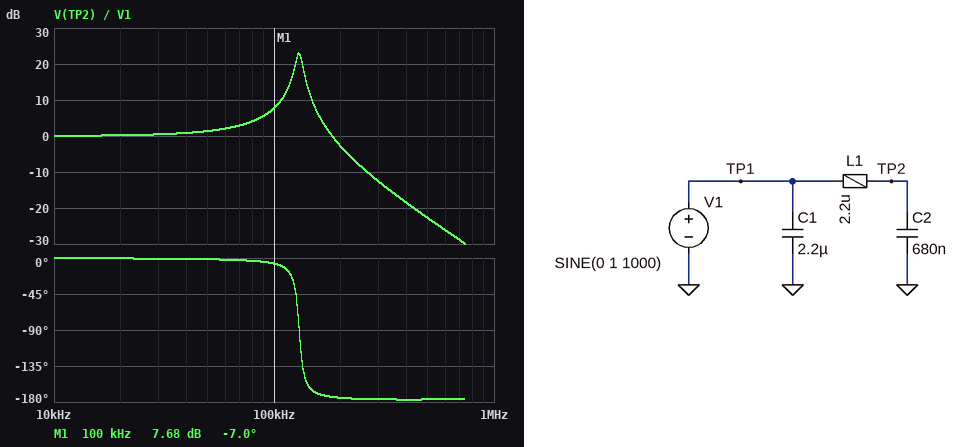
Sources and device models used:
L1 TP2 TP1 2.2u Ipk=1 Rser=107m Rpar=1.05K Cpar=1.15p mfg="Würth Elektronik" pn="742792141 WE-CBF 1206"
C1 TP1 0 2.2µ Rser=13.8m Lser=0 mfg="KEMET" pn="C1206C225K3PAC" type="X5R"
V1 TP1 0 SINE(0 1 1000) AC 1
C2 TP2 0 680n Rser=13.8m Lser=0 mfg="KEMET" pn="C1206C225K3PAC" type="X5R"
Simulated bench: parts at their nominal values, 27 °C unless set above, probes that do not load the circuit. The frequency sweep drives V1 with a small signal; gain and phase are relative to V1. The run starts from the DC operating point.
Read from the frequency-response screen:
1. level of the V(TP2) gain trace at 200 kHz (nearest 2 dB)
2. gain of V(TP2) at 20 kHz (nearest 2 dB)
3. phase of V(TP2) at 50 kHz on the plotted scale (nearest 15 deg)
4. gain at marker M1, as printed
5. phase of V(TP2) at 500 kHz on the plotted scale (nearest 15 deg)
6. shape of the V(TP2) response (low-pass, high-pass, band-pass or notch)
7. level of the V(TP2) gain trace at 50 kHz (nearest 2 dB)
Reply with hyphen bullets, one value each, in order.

- -2 dB
- 0 dB
- 0 deg
- 7.68 dB
- -180 deg
- low-pass
- 2 dB
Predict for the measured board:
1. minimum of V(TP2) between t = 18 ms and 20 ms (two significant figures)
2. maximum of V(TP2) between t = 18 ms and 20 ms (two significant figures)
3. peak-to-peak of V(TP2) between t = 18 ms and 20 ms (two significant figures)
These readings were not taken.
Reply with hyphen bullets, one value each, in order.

- -1.0 V
- 1.0 V
- 2.0 V
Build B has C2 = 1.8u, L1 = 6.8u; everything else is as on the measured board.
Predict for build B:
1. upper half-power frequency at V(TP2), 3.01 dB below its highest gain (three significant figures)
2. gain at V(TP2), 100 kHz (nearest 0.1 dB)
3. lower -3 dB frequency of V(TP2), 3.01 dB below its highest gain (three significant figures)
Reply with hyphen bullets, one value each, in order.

- 46.9 kHz
- -11.7 dB
- 44.0 kHz
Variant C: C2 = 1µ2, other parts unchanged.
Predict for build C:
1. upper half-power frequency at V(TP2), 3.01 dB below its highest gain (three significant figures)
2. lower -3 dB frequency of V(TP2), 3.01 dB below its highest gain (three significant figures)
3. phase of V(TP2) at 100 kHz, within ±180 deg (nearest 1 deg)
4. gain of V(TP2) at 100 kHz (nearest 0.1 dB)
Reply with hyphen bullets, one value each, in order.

- 102 kHz
- 93.2 kHz
- -114 deg
- 19.9 dB
